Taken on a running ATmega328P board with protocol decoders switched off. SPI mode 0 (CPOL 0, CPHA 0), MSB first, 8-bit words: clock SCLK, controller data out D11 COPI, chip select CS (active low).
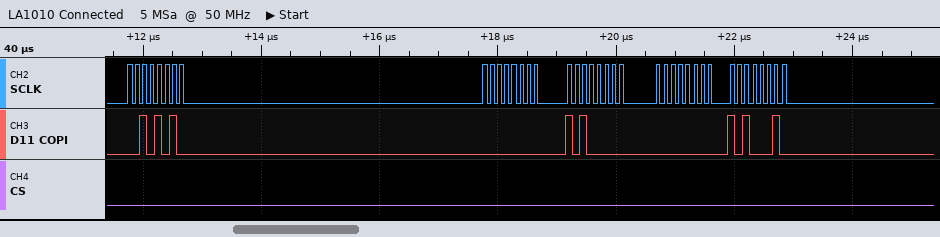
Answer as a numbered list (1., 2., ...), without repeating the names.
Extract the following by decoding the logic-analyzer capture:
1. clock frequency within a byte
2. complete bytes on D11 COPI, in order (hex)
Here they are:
1. 8 MHz
2. 0x2A 0x00 0xA0 0x00 0xA2
